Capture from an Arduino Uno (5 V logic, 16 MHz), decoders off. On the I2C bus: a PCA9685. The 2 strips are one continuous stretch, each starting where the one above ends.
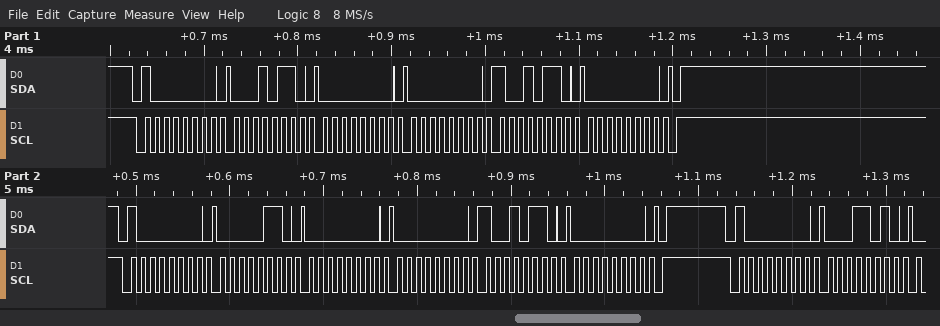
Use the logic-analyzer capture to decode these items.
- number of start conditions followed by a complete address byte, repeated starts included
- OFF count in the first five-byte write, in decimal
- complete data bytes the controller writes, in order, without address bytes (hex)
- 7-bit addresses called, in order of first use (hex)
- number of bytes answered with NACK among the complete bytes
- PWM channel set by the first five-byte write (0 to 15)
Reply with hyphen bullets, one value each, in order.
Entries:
- 3
- 150
- 16 00 00 96 00 06 00 00 96 00 1A
- 0x40
- 0
- 4
